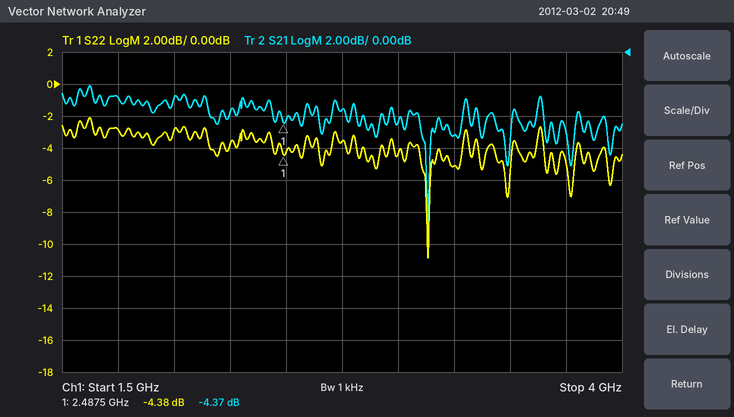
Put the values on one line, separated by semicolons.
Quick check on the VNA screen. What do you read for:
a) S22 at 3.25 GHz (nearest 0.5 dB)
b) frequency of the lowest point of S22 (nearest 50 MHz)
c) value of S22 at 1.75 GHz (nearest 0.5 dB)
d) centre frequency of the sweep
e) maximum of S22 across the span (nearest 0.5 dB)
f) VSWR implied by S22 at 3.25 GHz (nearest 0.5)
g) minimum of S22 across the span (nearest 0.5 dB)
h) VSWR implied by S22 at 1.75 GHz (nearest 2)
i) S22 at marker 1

-5.0 dB; 3.15 GHz; -3.0 dB; 2.75 GHz; -2.0 dB; 3.5; -11.0 dB; 6; -4.38 dB
